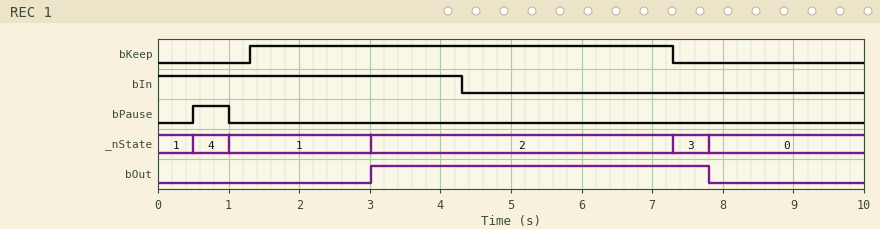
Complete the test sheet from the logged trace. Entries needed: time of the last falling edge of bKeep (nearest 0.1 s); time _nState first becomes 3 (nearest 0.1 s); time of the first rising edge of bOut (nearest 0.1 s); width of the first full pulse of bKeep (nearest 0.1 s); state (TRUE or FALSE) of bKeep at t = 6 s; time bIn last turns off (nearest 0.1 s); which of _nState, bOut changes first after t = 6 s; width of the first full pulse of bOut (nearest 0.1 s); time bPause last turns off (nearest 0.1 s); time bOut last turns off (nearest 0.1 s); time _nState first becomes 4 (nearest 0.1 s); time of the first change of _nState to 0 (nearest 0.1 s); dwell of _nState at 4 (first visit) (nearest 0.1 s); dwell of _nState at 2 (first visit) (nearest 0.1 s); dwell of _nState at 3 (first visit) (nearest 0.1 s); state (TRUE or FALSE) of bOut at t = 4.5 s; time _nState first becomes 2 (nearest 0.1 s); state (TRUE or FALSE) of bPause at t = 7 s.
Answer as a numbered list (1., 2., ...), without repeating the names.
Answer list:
1. 7.3 s
2. 7.3 s
3. 3.0 s
4. 6.0 s
5. TRUE
6. 4.3 s
7. _nState
8. 4.8 s
9. 1.0 s
10. 7.8 s
11. 0.5 s
12. 7.8 s
13. 0.5 s
14. 4.3 s
15. 0.5 s
16. TRUE
17. 3.0 s
18. FALSE
